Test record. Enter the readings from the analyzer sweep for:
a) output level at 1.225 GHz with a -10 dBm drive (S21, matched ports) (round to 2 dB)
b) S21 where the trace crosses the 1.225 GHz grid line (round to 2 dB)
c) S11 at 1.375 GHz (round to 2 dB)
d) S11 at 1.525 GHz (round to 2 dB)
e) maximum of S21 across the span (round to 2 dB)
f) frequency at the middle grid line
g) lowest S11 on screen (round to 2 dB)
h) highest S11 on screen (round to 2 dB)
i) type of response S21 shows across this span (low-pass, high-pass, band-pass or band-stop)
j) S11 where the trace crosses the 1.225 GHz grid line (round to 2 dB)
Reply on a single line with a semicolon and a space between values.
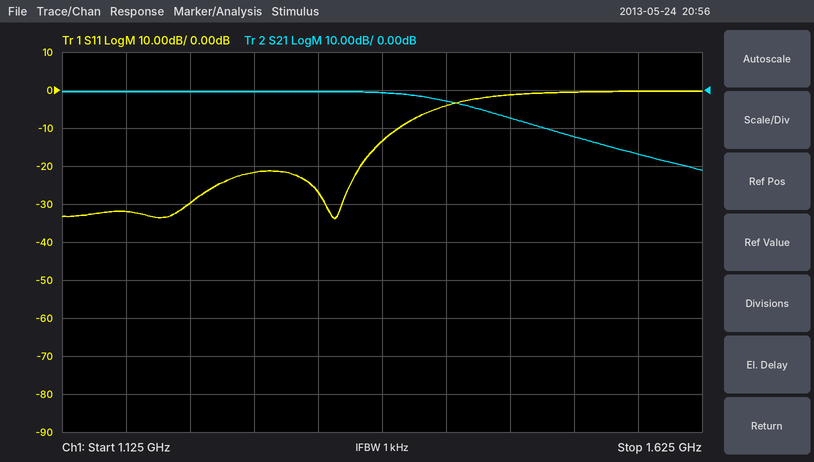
-10 dBm; 0 dB; -14 dB; 0 dB; 0 dB; 1.375 GHz; -34 dB; 0 dB; low-pass; -30 dB
